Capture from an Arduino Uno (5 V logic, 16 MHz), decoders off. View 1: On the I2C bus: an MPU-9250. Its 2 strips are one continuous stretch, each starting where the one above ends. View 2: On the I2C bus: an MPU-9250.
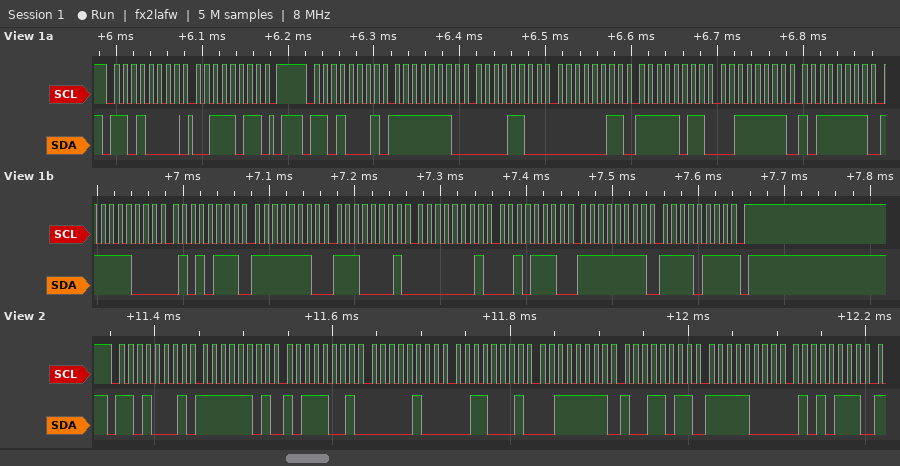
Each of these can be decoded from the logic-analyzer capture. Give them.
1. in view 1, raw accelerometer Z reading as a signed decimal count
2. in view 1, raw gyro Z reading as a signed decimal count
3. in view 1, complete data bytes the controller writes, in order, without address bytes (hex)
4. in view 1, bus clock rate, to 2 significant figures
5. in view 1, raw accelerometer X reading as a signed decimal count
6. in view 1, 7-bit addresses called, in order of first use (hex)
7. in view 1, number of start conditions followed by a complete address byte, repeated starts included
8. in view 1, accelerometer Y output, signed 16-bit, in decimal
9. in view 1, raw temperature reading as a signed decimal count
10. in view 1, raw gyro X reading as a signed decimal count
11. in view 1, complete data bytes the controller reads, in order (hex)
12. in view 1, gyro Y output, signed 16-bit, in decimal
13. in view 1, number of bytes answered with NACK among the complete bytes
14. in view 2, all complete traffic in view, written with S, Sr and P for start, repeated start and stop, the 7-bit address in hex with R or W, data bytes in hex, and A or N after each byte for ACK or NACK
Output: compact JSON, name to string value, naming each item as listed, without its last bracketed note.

{"in view 1, raw accelerometer Z reading as a signed decimal count": "16319", "in view 1, raw gyro Z reading as a signed decimal count": "-9", "in view 1, complete data bytes the controller writes, in order, without address bytes": "3B", "in view 1, bus clock rate, to 2 significant figures": "100 kHz", "in view 1, raw accelerometer X reading as a signed decimal count": "-500", "in view 1, 7-bit addresses called, in order of first use": "0x68", "in view 1, number of start conditions followed by a complete address byte, repeated starts included": "2", "in view 1, accelerometer Y output, signed 16-bit, in decimal": "1019", "in view 1, raw temperature reading as a signed decimal count": "-1961", "in view 1, raw gyro X reading as a signed decimal count": "-287", "in view 1, complete data bytes the controller reads, in order": "FE 0C 03 FB 3F BF F8 57 FE E1 01 2E FF F7", "in view 1, gyro Y output, signed 16-bit, in decimal": "302", "in view 1, number of bytes answered with NACK among the complete bytes": "1", "in view 2, all complete traffic in view, written with S, Sr and P for start, repeated start and stop, the 7-bit address in hex with R or W, data bytes in hex, and A or N after each byte for ACK or NACK": "S 68R A FD A B9 A 04 A 31 A 3F A 9B A F8 A 57 A"}
